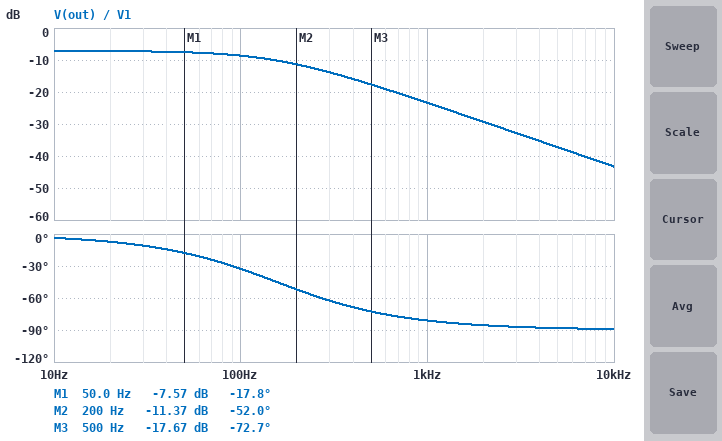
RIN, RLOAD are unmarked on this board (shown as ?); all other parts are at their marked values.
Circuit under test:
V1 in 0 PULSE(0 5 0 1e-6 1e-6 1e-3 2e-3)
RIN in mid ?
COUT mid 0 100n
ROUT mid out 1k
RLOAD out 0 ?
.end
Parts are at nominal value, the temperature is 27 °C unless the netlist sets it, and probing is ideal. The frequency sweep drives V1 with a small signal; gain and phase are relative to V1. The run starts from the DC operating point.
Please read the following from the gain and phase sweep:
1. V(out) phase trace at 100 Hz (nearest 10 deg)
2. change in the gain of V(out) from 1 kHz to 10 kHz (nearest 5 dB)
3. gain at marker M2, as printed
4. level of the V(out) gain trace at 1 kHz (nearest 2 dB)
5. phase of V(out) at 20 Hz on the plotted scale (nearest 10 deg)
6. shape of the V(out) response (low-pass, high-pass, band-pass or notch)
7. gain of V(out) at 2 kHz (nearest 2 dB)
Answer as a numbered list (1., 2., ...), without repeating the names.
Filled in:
1. -30 deg
2. -20 dB
3. -11.37 dB
4. -24 dB
5. -10 deg
6. low-pass
7. -30 dB
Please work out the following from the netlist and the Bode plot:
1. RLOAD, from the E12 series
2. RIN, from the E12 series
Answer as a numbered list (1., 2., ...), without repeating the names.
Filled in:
1. 18 kΩ
2. 22 kΩ
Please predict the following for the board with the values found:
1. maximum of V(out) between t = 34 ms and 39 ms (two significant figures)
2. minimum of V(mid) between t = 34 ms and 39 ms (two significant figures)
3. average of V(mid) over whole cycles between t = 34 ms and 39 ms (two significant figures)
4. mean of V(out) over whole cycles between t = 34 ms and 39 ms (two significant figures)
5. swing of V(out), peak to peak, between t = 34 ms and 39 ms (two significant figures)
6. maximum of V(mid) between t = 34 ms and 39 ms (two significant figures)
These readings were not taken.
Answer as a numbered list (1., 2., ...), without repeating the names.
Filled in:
1. 1.6 V
2. 630 mV
3. 1.2 V
4. 1.1 V
5. 1.0 V
6. 1.7 V
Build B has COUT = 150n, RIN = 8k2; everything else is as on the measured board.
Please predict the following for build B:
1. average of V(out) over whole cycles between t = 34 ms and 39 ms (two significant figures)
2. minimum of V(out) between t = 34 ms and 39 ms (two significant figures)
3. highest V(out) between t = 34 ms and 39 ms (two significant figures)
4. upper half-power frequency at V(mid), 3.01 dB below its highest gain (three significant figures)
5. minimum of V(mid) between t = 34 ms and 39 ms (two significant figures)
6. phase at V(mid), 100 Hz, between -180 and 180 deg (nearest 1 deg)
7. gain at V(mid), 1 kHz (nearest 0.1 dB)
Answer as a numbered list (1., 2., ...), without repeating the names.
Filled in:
1. 1.7 V
2. 790 mV
3. 2.5 V
4. 185 Hz
5. 830 mV
6. -28 deg
7. -17.9 dB
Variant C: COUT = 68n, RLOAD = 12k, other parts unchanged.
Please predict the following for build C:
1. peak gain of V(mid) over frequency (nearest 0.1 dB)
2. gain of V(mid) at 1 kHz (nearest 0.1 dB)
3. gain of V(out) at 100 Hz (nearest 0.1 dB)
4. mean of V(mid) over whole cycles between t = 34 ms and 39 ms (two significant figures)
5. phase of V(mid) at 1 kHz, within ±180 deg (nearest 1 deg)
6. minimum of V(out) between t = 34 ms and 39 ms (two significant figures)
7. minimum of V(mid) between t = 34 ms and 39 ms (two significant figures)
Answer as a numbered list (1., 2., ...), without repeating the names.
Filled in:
1. -8.6 dB
2. -19.8 dB
3. -9.8 dB
4. 930 mV
5. -74 deg
6. 240 mV
7. 260 mV
